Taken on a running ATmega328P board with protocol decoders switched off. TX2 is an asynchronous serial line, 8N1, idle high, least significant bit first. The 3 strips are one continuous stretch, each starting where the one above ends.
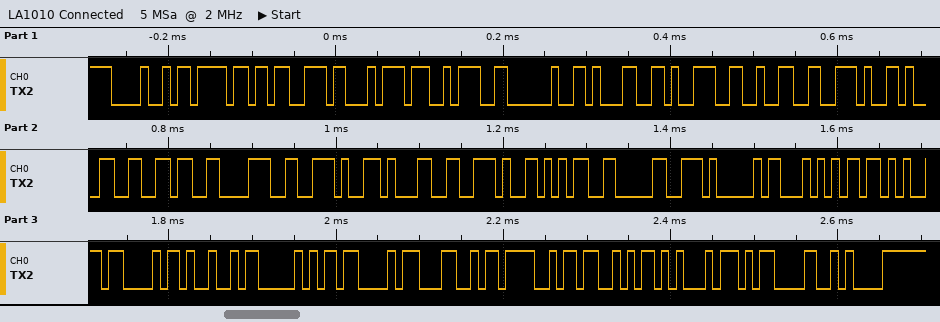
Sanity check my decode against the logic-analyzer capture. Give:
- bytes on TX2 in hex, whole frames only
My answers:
0x48 0x6F 0x73 0x74 0x3A 0x20 0x31 0x39 0x32 0x2E 0x31 0x36 0x38 0x2E 0x31 0x2E 0x35 0x30 0x41 0x54 0x2B 0x43 0x49 0x50 0x43 0x4C 0x4F 0x53 0x45 0x0D 0x0A
